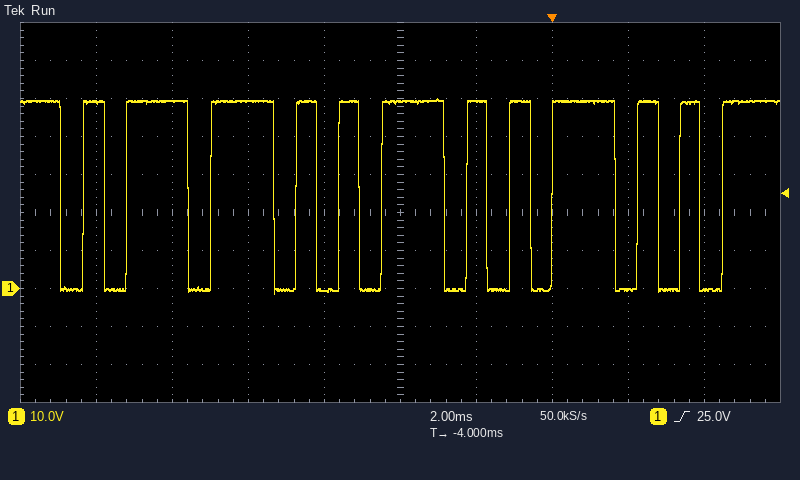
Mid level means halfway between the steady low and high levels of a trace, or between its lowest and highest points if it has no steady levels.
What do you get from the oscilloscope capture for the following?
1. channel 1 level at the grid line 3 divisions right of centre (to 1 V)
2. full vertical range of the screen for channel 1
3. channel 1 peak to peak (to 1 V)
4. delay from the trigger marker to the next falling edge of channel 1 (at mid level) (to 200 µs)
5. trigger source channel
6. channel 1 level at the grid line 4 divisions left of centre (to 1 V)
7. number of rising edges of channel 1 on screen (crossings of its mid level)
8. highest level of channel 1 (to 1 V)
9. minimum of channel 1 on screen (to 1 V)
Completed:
0 V
100 V
51 V
1.6 ms
channel 1
49 V
12
50 V
-1 V
